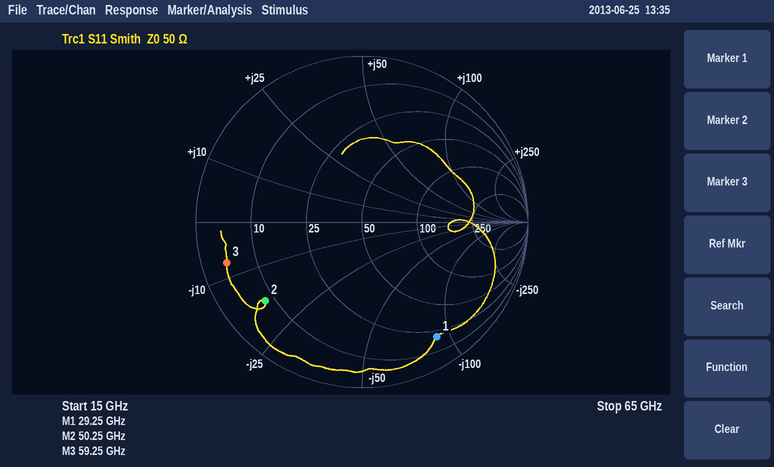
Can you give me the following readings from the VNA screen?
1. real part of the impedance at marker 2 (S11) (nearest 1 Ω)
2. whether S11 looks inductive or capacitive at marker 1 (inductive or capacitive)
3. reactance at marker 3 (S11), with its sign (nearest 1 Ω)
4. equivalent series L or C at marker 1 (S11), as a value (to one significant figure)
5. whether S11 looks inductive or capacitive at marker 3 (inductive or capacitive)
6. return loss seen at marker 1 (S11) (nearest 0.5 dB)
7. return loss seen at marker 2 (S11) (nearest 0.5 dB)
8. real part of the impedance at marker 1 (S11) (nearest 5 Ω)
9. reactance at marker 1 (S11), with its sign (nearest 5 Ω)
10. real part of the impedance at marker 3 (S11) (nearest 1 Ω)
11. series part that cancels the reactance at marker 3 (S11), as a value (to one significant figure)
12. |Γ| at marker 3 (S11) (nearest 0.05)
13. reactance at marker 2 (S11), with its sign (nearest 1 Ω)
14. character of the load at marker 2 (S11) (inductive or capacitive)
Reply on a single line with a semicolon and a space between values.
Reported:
8 Ω; capacitive; -7 Ω; 60 fF; capacitive; 1.5 dB; 2.5 dB; 20 Ω; -90 Ω; 4 Ω; 20 pH; 0.85; -17 Ω; capacitive
